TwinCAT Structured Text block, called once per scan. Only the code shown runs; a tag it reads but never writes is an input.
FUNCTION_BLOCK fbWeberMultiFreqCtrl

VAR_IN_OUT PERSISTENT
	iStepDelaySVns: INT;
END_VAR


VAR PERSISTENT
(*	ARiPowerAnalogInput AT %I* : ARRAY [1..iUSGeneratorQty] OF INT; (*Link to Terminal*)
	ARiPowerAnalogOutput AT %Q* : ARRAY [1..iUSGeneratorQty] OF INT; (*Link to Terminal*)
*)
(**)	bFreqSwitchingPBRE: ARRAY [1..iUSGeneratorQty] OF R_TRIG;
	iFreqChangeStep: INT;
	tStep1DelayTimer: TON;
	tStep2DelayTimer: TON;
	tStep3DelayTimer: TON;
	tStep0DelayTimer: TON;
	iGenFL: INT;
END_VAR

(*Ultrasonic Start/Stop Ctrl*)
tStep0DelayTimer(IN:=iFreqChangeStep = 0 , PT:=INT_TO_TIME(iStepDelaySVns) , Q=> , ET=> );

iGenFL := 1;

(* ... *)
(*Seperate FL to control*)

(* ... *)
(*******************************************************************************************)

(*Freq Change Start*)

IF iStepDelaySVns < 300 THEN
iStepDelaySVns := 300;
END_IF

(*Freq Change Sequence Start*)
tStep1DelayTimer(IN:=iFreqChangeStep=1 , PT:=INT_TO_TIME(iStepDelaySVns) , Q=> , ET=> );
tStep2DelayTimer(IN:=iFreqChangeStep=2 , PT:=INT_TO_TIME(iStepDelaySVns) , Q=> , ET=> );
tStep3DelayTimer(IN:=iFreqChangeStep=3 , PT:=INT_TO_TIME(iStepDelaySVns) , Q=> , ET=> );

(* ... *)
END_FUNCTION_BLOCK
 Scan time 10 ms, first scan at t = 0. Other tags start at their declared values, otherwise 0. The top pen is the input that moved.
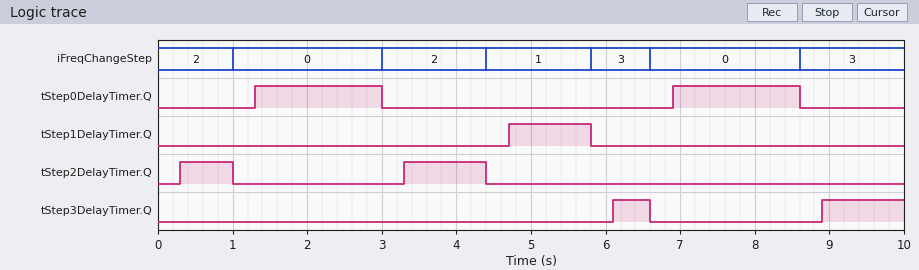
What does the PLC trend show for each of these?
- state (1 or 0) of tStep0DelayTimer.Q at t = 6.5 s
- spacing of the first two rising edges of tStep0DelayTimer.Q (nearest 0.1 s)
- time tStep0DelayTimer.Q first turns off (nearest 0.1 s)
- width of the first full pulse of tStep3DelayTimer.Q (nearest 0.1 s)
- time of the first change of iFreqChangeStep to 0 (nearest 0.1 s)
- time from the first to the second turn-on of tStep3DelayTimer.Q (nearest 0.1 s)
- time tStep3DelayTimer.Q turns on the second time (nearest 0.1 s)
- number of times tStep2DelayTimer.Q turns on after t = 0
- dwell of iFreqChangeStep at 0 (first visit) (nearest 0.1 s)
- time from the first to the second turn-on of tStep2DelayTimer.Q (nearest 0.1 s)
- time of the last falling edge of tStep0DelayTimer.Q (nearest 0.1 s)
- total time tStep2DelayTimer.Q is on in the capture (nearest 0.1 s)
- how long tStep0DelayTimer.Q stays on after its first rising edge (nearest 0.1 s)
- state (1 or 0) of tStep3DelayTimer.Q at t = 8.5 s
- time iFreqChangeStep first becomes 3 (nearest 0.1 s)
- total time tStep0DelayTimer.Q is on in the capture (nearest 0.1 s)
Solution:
0
5.6 s
3.0 s
0.5 s
1.0 s
2.8 s
8.9 s
2
2.0 s
3.0 s
8.6 s
1.8 s
1.7 s
0
5.8 s
3.4 s
